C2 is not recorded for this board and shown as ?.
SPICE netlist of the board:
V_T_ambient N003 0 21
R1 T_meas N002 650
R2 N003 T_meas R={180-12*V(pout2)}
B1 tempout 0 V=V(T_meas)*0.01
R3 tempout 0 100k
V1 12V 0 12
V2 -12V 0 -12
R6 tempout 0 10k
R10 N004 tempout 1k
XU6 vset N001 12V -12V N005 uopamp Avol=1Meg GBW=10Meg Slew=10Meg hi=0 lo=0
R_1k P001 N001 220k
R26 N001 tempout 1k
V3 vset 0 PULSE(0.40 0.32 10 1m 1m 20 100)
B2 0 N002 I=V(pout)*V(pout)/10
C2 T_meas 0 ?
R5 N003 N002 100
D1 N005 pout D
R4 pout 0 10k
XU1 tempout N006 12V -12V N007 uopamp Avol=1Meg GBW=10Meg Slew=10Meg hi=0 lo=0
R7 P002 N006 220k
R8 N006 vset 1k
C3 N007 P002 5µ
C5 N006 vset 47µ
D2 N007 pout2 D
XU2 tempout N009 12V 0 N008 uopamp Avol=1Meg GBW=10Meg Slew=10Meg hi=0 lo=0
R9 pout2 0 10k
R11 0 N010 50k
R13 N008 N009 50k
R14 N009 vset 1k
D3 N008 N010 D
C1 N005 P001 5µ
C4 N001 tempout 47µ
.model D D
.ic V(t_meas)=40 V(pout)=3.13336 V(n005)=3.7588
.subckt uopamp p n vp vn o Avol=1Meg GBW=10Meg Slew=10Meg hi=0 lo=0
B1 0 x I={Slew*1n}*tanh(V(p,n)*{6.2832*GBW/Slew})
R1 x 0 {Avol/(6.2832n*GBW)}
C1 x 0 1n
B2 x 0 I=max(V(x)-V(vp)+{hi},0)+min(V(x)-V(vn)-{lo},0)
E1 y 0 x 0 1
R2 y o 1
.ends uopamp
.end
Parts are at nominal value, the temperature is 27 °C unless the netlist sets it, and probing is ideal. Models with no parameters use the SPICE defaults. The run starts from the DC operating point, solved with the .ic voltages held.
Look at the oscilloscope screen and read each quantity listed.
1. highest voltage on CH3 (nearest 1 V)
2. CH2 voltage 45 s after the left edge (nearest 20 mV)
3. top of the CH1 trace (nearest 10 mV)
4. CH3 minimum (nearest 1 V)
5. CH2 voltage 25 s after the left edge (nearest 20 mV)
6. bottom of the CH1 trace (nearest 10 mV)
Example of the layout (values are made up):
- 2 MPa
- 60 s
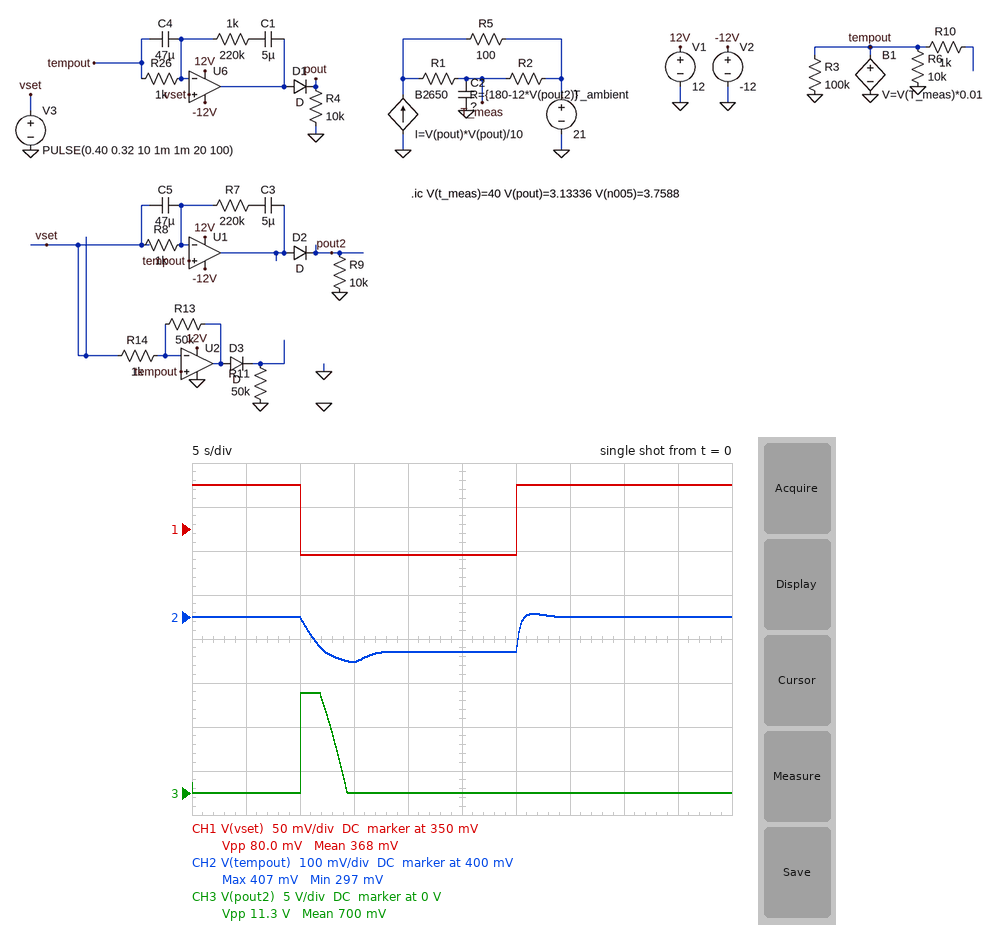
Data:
- 11 V
- 400 mV
- 400 mV
- 0 V
- 320 mV
- 320 mV
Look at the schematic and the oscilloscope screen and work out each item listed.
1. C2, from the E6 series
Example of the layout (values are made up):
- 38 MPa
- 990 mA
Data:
- 100 mF
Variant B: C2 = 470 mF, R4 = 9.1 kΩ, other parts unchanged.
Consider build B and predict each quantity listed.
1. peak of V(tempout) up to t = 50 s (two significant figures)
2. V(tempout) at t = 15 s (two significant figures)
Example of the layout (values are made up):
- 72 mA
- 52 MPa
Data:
- 420 mV
- 360 mV
